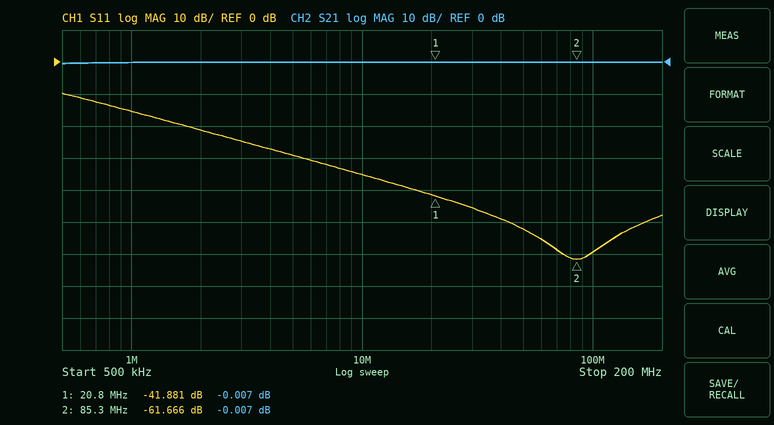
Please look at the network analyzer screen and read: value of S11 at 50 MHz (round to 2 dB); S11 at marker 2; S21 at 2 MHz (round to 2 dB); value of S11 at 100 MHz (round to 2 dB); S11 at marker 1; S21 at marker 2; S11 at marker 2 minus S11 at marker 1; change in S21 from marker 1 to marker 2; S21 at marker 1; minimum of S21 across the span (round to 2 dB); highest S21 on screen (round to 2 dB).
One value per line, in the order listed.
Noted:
-52 dB
-61.666 dB
0 dB
-60 dB
-41.881 dB
-0.007 dB
-19.785 dB
0.000 dB
-0.007 dB
0 dB
0 dB
